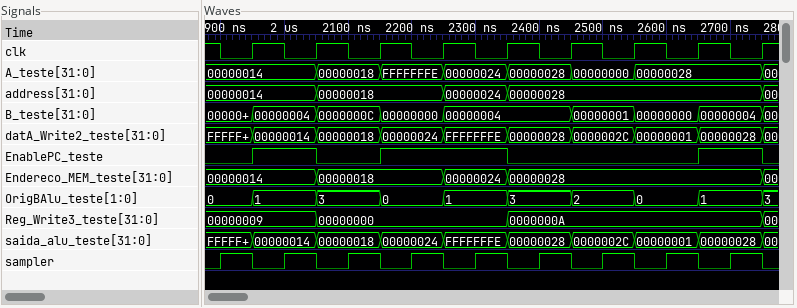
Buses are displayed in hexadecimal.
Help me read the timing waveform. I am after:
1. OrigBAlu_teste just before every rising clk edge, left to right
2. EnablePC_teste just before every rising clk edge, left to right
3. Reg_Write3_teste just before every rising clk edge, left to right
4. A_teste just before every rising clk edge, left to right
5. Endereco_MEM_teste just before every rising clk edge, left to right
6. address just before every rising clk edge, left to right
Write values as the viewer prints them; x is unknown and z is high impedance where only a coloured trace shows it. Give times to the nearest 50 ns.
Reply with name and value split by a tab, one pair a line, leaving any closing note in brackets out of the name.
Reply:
OrigBAlu_teste just before every rising clk edge, left to right	0, 1, 3, 0, 1, 3, 2, 0, 1
EnablePC_teste just before every rising clk edge, left to right	0 1 0 1 1 0 0 0 1
Reg_Write3_teste just before every rising clk edge, left to right	00000009, 00000009, 00000000, 00000000, 00000000, 0000000A, 0000000A, 0000000A, 0000000A
A_teste just before every rising clk edge, left to right	00000014, 00000014, 00000018, FFFFFFFE, 00000024, 00000028, 00000000, 00000028, 00000028
Endereco_MEM_teste just before every rising clk edge, left to right	00000014, 00000014, 00000018, 00000018, 00000024, 00000028, 00000028, 00000028, 00000028
address just before every rising clk edge, left to right	00000014, 00000014, 00000018, 00000018, 00000024, 00000028, 00000028, 00000028, 00000028
